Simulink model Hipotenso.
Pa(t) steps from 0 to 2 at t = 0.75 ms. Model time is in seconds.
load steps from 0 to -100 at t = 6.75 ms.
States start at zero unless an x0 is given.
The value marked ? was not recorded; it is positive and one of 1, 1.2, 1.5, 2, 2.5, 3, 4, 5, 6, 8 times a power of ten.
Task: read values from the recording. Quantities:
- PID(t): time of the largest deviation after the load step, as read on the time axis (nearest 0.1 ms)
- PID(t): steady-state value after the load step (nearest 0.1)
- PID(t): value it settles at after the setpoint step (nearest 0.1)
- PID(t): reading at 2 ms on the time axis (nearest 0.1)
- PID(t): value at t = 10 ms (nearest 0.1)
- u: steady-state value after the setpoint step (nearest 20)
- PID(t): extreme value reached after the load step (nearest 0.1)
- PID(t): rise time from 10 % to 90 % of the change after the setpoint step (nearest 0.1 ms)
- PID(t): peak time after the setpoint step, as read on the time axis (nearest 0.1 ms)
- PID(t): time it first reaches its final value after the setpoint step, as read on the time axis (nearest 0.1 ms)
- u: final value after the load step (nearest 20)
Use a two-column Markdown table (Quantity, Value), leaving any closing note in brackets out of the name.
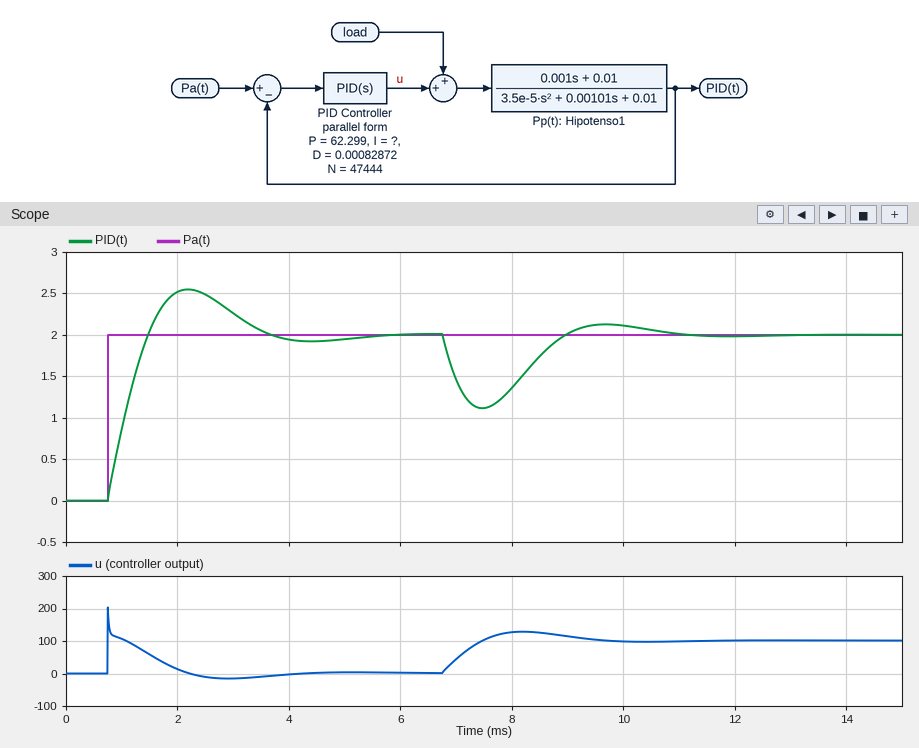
| Quantity | Value |
|---|---|
| PID(t): time of the largest deviation after the load step, as read on the time axis | 7.5 ms |
| PID(t): steady-state value after the load step | 2.0 |
| PID(t): value it settles at after the setpoint step | 2.0 |
| PID(t): reading at 2 ms on the time axis | 2.5 |
| PID(t): value at t = 10 ms | 2.1 |
| u: steady-state value after the setpoint step | 0 |
| PID(t): extreme value reached after the load step | 1.1 |
| PID(t): rise time from 10 % to 90 % of the change after the setpoint step | 0.6 ms |
| PID(t): peak time after the setpoint step, as read on the time axis | 2.2 ms |
| PID(t): time it first reaches its final value after the setpoint step, as read on the time axis | 1.5 ms |
| u: final value after the load step | 100 |
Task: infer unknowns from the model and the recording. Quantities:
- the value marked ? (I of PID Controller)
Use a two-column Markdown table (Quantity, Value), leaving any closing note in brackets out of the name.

| Quantity | Value |
|---|---|
| the value marked ? | 100000 |
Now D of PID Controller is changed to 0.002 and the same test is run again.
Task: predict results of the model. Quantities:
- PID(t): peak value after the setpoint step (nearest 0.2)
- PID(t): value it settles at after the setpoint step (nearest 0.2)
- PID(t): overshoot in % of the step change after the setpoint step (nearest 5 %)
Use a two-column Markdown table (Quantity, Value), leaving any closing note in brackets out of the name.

| Quantity | Value |
|---|---|
| PID(t): peak value after the setpoint step | 2.6 |
| PID(t): value it settles at after the setpoint step | 2.0 |
| PID(t): overshoot in % of the step change after the setpoint step | 25 % |
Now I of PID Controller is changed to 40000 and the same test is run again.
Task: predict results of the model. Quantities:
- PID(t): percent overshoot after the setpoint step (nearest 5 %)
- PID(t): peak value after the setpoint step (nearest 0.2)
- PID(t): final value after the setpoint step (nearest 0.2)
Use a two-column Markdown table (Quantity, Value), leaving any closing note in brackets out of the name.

| Quantity | Value |
|---|---|
| PID(t): percent overshoot after the setpoint step | 15 % |
| PID(t): peak value after the setpoint step | 2.4 |
| PID(t): final value after the setpoint step | 2.0 |
